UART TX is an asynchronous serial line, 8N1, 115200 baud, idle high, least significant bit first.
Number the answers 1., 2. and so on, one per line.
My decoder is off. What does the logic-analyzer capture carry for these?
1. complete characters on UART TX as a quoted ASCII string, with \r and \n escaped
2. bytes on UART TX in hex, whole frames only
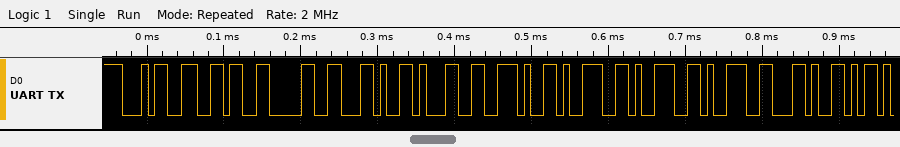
1. "460,1.999,"
2. 0x34 0x36 0x30 0x2C 0x31 0x2E 0x39 0x39 0x39 0x2C
